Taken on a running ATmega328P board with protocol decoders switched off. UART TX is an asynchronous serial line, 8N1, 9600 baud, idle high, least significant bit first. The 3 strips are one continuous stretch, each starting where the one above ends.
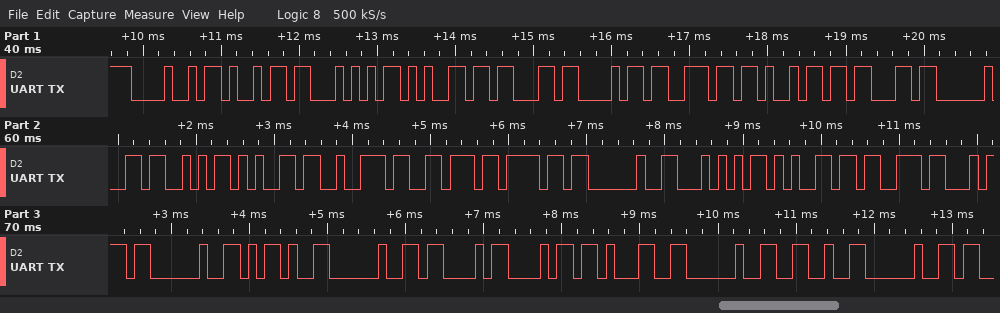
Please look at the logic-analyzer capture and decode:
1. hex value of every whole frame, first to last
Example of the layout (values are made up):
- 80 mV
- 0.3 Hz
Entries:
- 48 69 54 65 63 68 6E 69 63 20 53 65 72 76 6F 20 54 65 73 74 20 2D 20 43 68 31 20 26 20
